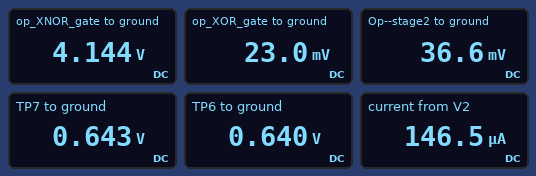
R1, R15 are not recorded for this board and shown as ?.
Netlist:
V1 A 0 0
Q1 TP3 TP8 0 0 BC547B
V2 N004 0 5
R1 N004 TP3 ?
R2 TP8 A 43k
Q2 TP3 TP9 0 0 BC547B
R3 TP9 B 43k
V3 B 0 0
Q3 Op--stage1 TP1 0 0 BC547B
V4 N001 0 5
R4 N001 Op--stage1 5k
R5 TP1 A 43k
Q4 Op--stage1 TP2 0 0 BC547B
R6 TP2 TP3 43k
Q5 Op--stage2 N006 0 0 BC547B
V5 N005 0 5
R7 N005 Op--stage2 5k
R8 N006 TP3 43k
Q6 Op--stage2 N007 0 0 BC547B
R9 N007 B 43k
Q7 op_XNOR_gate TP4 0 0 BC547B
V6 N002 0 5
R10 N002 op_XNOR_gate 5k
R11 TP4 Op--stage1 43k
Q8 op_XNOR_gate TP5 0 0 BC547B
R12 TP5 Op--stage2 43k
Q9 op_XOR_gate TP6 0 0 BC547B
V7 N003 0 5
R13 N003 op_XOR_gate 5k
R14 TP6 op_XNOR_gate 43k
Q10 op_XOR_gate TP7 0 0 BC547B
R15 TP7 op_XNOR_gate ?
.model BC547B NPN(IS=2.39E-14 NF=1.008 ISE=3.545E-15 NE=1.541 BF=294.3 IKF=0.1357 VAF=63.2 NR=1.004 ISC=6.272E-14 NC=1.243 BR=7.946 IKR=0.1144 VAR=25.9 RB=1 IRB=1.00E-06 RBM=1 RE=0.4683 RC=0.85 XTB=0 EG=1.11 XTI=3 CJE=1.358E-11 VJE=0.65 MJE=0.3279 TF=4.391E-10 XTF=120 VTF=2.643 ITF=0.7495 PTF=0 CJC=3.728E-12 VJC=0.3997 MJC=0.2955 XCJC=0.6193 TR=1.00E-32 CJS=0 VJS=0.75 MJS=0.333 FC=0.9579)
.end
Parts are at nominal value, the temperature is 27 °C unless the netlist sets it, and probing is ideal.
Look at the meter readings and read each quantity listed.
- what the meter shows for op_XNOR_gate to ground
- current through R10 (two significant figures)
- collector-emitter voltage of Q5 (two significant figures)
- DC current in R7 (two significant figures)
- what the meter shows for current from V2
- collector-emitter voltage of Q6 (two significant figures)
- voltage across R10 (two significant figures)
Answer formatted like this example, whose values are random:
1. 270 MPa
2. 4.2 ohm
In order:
1. 4.144 V
2. 170 µA
3. 37 mV
4. 990 µA
5. 146.5 µA
6. 37 mV
7. 860 mV
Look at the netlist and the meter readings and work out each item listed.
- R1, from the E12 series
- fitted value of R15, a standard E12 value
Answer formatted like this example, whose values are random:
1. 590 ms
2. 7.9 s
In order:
1. 8.2 kΩ
2. 39 kΩ
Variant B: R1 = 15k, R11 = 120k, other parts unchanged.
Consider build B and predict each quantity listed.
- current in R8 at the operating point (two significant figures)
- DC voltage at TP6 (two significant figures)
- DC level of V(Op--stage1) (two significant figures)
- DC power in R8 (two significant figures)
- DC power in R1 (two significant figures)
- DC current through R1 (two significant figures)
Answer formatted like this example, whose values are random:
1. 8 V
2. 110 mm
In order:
1. 60 µA
2. 640 mV
3. 41 mV
4. 150 µW
5. 210 µW
6. 120 µA
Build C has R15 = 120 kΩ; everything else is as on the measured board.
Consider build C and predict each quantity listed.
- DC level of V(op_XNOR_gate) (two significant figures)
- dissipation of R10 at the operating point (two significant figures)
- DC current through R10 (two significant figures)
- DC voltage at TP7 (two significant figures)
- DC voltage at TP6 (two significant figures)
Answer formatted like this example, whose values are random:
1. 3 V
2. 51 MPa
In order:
1. 4.4 V
2. 71 µW
3. 120 µA
4. 620 mV
5. 650 mV
